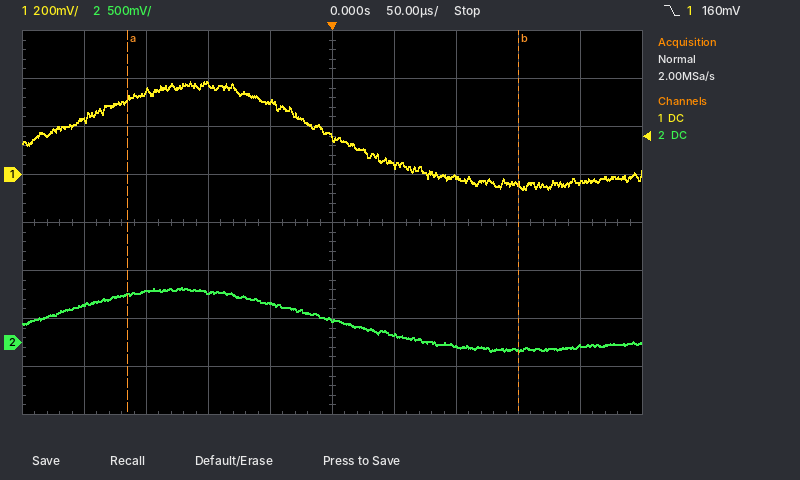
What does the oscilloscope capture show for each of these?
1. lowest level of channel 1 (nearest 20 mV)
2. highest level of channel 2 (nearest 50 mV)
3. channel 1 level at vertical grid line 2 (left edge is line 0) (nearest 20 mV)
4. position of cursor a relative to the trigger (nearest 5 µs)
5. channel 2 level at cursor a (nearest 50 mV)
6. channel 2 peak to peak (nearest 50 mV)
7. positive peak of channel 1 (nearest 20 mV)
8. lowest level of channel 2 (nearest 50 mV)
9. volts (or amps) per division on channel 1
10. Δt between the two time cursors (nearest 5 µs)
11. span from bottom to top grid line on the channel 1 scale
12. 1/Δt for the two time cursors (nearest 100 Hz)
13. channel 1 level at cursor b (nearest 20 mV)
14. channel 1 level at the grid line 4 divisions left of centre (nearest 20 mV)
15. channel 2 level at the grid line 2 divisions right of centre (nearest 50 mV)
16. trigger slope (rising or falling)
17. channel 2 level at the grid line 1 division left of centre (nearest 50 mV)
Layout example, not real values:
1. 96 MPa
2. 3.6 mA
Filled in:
1. -60 mV
2. 550 mV
3. 340 mV
4. -165 µs
5. 500 mV
6. 650 mV
7. 380 mV
8. -100 mV
9. 200 mV
10. 315 µs
11. 1.6 V
12. 3.2 kHz
13. -40 mV
14. 220 mV
15. -50 mV
16. falling
17. 400 mV
